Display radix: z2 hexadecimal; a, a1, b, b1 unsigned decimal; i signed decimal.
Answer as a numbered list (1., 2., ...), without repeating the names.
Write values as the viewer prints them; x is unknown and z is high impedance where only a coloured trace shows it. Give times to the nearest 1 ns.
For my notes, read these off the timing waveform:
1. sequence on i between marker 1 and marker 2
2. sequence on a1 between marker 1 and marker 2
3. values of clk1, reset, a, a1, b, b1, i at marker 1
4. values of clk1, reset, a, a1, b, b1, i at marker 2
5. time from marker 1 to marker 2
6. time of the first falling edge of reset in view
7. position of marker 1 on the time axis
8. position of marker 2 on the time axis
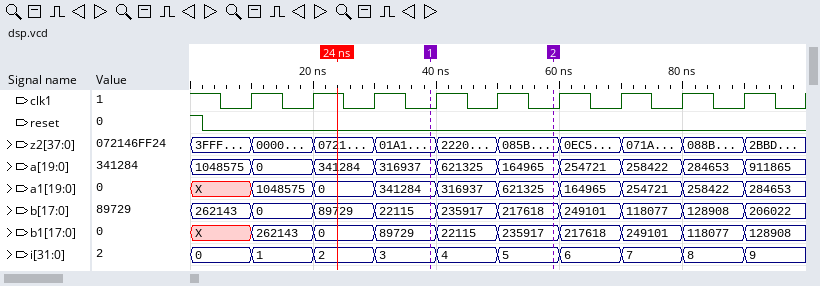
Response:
1. 3, 4, 5
2. 341284, 316937, 621325
3. clk1=0, reset=0, a=316937, a1=341284, b=22115, b1=89729, i=3
4. clk1=0, reset=0, a=164965, a1=621325, b=217618, b1=235917, i=5
5. 20 ns
6. 2 ns
7. 39 ns
8. 59 ns
